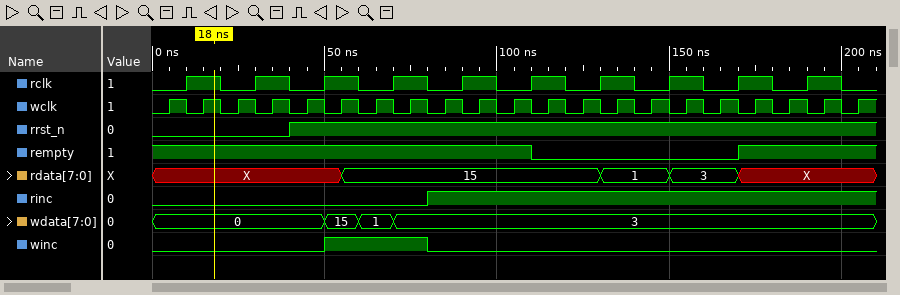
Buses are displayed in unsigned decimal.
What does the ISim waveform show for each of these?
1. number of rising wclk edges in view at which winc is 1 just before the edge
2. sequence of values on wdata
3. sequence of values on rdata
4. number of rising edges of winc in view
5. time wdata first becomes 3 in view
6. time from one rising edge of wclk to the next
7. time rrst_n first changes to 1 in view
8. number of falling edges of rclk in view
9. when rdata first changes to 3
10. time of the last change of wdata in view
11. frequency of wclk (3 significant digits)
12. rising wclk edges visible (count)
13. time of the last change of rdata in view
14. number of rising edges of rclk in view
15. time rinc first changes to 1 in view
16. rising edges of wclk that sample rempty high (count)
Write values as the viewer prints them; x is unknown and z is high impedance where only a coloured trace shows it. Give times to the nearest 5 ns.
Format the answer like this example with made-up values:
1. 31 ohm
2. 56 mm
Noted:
1. 3
2. 0, 15, 1, 3
3. X, 15, 1, 3, X
4. 1
5. 70 ns
6. 10 ns
7. 40 ns
8. 10
9. 150 ns
10. 70 ns
11. 100 MHz
12. 21
13. 170 ns
14. 10
15. 80 ns
16. 15
